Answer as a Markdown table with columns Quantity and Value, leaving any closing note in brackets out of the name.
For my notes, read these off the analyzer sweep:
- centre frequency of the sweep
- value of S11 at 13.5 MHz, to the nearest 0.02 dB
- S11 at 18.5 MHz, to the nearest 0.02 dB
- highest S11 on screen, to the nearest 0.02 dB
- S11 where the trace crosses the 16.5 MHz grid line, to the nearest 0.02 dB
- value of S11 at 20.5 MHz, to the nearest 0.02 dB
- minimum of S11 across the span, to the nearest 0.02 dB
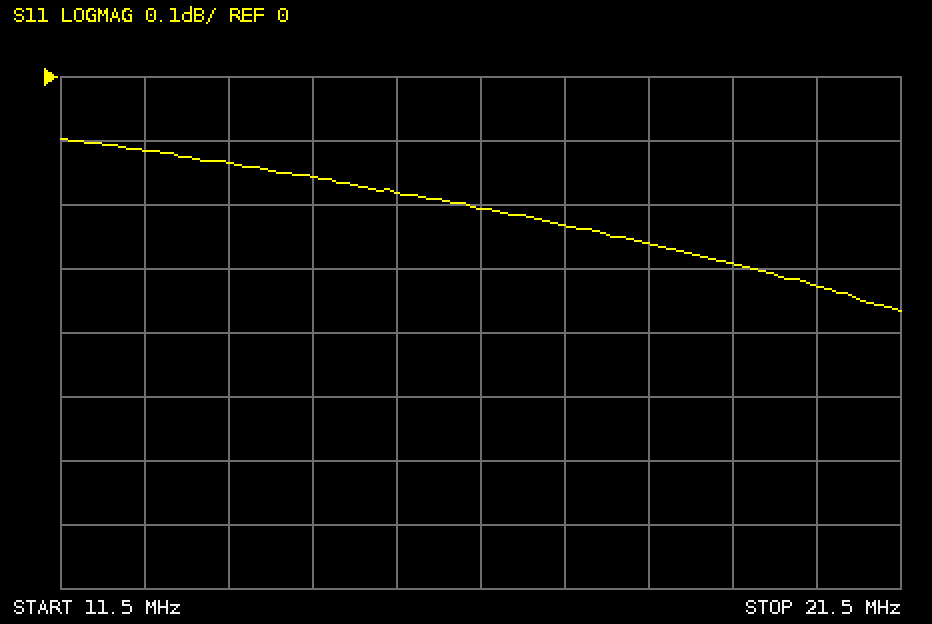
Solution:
| Quantity | Value |
|---|---|
| centre frequency of the sweep | 16.5 MHz |
| value of S11 at 13.5 MHz, to the nearest 0.02 dB | -0.14 dB |
| S11 at 18.5 MHz, to the nearest 0.02 dB | -0.26 dB |
| highest S11 on screen, to the nearest 0.02 dB | -0.10 dB |
| S11 where the trace crosses the 16.5 MHz grid line, to the nearest 0.02 dB | -0.20 dB |
| value of S11 at 20.5 MHz, to the nearest 0.02 dB | -0.32 dB |
| minimum of S11 across the span, to the nearest 0.02 dB | -0.36 dB |
